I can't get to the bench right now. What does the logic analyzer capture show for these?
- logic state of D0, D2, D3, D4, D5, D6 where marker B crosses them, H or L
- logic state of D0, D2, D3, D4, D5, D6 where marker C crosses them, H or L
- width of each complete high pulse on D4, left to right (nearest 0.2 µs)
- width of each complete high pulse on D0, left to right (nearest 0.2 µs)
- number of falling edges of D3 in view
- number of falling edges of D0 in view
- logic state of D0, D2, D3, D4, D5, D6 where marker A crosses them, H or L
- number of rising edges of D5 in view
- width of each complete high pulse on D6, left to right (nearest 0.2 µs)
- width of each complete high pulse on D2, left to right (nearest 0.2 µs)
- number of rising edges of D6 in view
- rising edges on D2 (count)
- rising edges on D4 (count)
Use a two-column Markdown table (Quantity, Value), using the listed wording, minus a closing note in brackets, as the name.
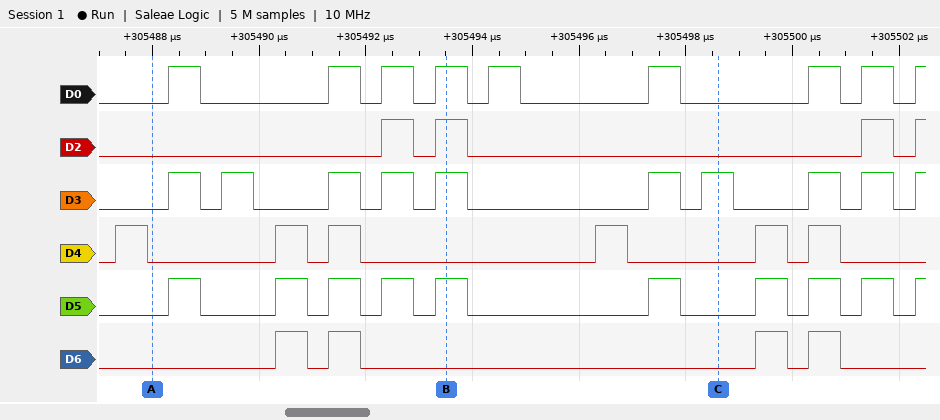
| Quantity | Value |
|---|---|
| logic state of D0, D2, D3, D4, D5, D6 where marker B crosses them, H or L | D0=H, D2=H, D3=H, D4=L, D5=H, D6=L |
| logic state of D0, D2, D3, D4, D5, D6 where marker C crosses them, H or L | D0=L, D2=L, D3=H, D4=L, D5=L, D6=L |
| width of each complete high pulse on D4, left to right | 0.6 µs, 0.6 µs, 0.6 µs, 0.6 µs, 0.6 µs, 0.6 µs |
| width of each complete high pulse on D0, left to right | 0.6 µs, 0.6 µs, 0.6 µs, 0.6 µs, 0.6 µs, 0.6 µs, 0.6 µs, 0.6 µs |
| number of falling edges of D3 in view | 9 |
| number of falling edges of D0 in view | 8 |
| logic state of D0, D2, D3, D4, D5, D6 where marker A crosses them, H or L | D0=L, D2=L, D3=L, D4=L, D5=L, D6=L |
| number of rising edges of D5 in view | 10 |
| width of each complete high pulse on D6, left to right | 0.6 µs, 0.6 µs, 0.6 µs, 0.6 µs |
| width of each complete high pulse on D2, left to right | 0.6 µs, 0.6 µs, 0.6 µs |
| number of rising edges of D6 in view | 4 |
| rising edges on D2 | 4 |
| rising edges on D4 | 6 |
